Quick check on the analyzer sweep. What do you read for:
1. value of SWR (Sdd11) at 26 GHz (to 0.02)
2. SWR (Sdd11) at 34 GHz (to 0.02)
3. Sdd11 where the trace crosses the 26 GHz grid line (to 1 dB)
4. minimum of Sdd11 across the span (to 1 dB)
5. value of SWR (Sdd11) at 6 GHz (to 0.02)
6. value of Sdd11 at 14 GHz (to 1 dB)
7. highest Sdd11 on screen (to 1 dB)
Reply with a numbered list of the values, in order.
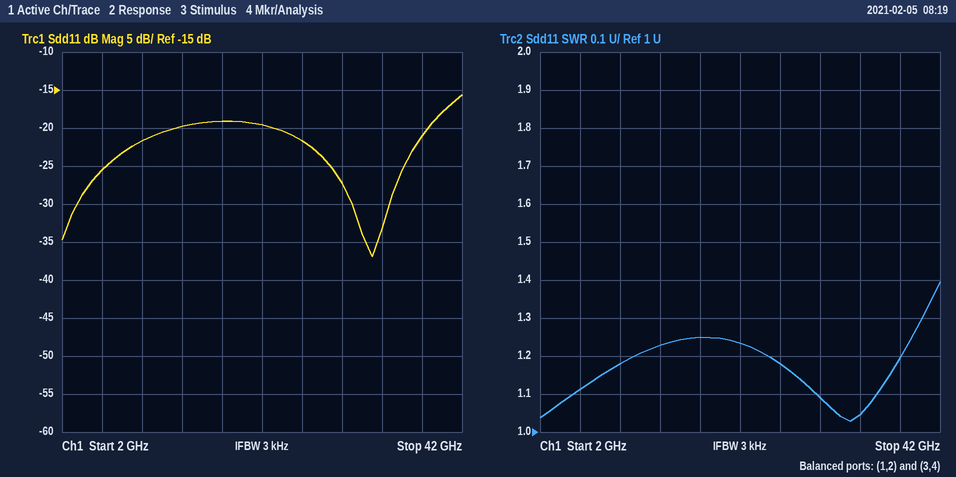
1. 1.18
2. 1.04
3. -22 dB
4. -37 dB
5. 1.12
6. -20 dB
7. -16 dB
